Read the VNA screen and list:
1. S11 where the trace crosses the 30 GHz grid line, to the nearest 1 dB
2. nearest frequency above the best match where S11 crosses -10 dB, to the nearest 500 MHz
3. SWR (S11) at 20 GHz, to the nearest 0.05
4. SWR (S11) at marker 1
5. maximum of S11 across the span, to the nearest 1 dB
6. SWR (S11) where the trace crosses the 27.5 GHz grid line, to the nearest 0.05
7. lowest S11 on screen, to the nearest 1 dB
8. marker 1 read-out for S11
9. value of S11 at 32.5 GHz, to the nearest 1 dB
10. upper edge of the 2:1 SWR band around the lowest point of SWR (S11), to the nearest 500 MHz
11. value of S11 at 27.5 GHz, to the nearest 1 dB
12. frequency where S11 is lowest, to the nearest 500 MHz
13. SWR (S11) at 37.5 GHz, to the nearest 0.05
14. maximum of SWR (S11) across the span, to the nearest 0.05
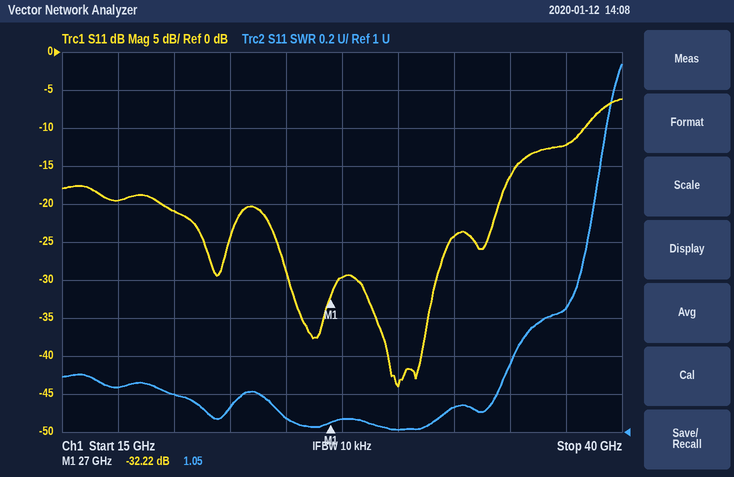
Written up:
-44 dB
38.5 GHz
1.20
1.05
-6 dB
1.05
-44 dB
-32.22 dB
-24 dB
38.5 GHz
-30 dB
30.0 GHz
1.65
2.95
